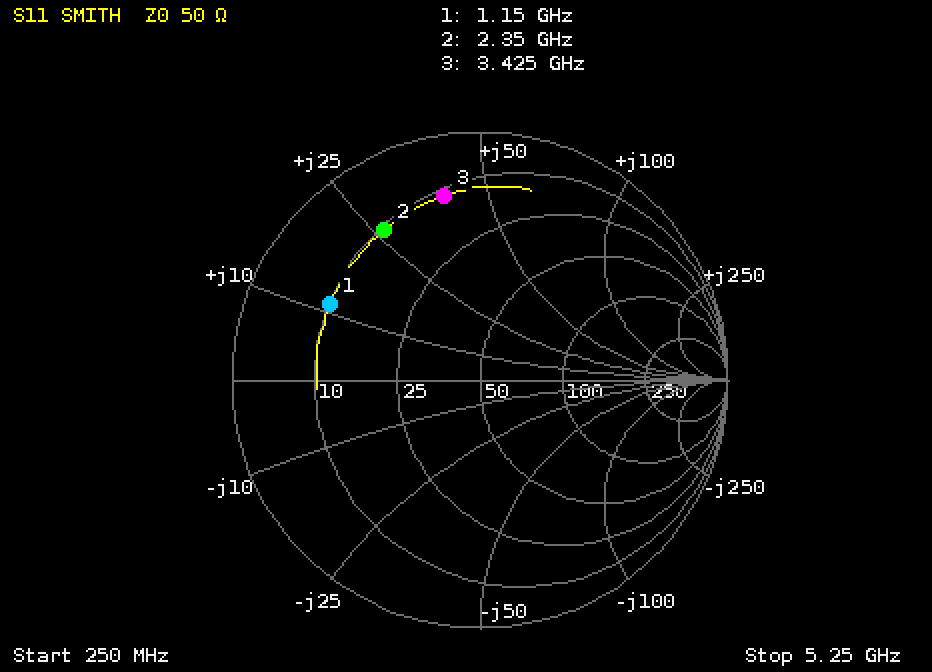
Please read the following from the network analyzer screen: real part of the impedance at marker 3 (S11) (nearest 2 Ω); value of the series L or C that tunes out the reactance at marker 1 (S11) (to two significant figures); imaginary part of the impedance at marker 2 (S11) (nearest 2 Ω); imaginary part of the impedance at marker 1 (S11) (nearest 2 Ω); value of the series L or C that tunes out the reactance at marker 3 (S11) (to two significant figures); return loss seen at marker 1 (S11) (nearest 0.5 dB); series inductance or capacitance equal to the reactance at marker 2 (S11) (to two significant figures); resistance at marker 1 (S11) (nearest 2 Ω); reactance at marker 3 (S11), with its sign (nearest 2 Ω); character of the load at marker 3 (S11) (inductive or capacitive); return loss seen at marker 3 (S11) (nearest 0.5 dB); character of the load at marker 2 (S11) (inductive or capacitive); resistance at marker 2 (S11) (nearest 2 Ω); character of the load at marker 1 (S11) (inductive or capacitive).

12 Ω
12 pF
+26 Ω
+12 Ω
1.2 pF
3.5 dB
1.8 nH
10 Ω
+40 Ω
inductive
2.5 dB
inductive
10 Ω
inductive
